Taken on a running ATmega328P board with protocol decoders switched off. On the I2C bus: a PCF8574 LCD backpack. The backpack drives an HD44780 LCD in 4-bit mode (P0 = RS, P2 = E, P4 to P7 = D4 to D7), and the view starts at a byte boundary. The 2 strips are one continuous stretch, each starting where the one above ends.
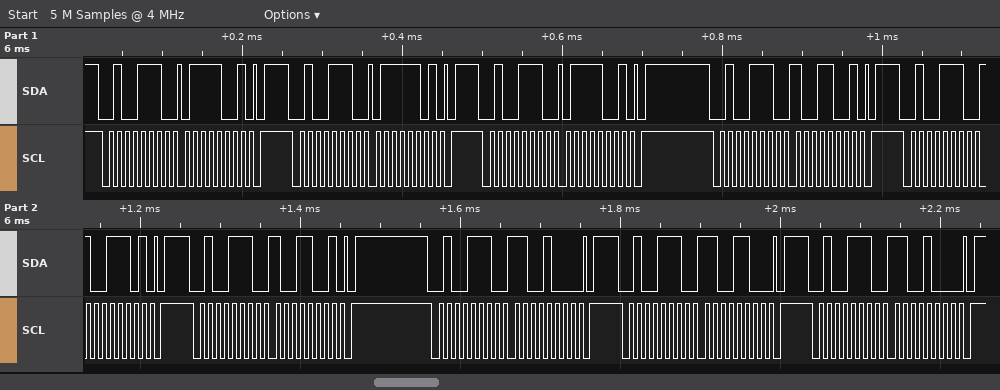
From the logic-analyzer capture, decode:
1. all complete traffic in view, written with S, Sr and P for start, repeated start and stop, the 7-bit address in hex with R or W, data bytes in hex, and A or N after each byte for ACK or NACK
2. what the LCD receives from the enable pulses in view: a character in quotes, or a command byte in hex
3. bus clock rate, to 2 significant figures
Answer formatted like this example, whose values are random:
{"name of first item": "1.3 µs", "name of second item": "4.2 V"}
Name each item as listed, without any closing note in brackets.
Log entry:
{"all complete traffic in view, written with S, Sr and P for start, repeated start and stop, the 7-bit address in hex with R or W, data bytes in hex, and A or N after each byte for ACK or NACK": "S 27W A 79 A P S 27W A 7D A P S 27W A 79 A P S 27W A 99 A P S 27W A 9D A P S 27W A 99 A P S 27W A C8 A P S 27W A CC A P S 27W A C8 A P", "what the LCD receives from the enable pulses in view: a character in quotes, or a command byte in hex": "'y'", "bus clock rate, to 2 significant figures": "100 kHz"}
